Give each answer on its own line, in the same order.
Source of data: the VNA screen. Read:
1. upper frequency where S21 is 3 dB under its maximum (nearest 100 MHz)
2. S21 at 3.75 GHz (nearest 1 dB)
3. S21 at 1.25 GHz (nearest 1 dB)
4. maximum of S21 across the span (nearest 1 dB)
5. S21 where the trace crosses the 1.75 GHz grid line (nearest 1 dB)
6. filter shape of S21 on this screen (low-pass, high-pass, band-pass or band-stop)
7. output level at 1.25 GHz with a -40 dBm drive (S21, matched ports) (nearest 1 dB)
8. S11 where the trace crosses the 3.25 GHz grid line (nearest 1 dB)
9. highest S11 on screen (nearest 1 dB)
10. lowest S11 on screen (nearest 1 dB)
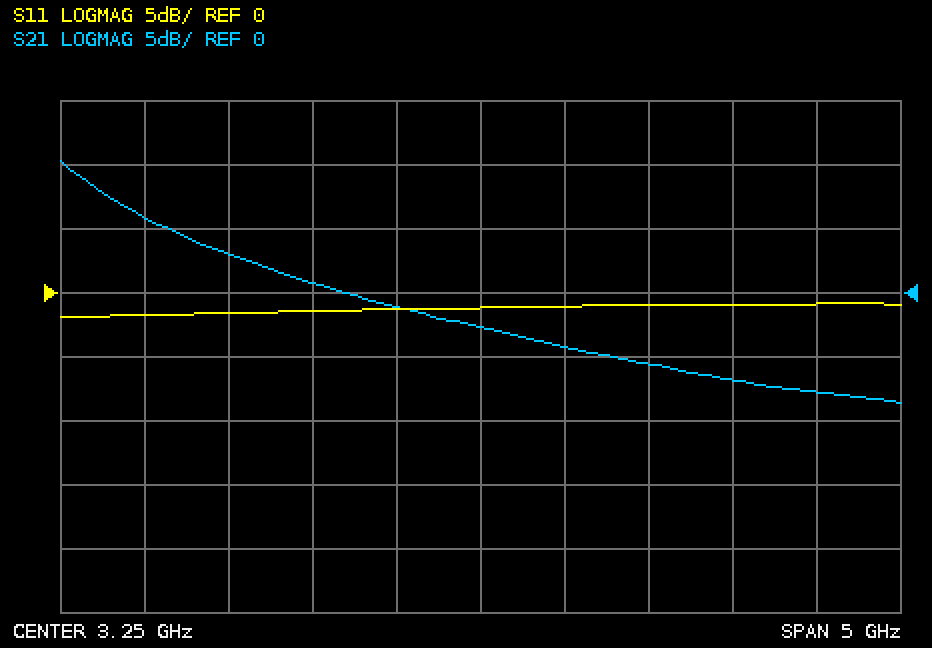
1.1 GHz
-4 dB
6 dB
10 dB
3 dB
low-pass
-34 dBm
-1 dB
-1 dB
-2 dB
